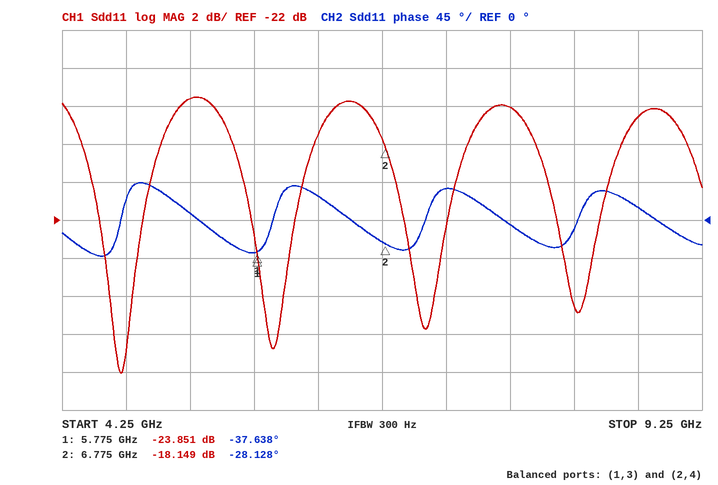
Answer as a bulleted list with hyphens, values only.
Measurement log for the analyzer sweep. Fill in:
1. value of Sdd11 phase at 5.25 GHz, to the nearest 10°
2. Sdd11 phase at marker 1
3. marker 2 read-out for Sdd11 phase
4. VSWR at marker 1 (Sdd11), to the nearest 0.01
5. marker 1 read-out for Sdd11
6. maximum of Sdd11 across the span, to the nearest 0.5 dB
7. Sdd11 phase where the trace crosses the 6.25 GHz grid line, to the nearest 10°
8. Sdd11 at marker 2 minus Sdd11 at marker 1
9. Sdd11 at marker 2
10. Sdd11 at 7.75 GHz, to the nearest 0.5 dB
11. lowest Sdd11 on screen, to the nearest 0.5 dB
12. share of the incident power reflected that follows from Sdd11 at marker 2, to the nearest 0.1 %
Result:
- 10°
- -37.638°
- -28.128°
- 1.14
- -23.851 dB
- -15.5 dB
- 30°
- 5.702 dB
- -18.149 dB
- -16.0 dB
- -30.0 dB
- 1.5 %
